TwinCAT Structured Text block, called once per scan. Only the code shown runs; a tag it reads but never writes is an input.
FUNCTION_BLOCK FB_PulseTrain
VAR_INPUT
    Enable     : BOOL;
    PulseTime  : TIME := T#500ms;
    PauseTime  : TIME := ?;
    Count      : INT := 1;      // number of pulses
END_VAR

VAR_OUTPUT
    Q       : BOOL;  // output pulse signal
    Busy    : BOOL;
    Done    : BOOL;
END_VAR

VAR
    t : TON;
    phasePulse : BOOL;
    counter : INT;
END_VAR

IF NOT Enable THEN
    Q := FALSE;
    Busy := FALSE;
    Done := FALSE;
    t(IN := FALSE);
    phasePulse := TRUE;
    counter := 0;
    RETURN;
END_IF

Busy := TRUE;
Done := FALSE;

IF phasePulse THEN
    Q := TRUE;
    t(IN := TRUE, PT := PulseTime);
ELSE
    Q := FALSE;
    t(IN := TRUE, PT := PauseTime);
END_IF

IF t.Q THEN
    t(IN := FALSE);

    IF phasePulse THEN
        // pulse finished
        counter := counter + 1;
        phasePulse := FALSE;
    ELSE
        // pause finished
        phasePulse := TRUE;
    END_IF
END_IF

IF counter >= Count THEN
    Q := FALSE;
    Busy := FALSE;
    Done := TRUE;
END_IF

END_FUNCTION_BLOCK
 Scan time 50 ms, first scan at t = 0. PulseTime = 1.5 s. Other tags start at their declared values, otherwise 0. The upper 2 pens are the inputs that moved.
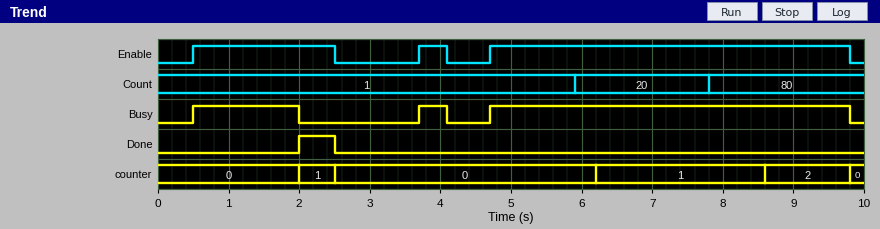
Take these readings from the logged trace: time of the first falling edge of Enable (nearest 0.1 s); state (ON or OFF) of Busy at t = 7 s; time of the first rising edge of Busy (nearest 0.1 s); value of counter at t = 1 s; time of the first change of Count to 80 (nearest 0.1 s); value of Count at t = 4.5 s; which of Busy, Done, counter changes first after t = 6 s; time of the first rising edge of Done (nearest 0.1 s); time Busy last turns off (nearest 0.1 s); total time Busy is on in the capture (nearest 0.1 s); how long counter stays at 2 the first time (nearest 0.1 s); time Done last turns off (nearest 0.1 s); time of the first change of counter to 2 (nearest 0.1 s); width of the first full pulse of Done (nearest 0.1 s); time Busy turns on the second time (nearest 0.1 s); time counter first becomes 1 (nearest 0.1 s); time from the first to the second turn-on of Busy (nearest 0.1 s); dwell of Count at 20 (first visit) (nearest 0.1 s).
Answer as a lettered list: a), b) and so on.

a) 2.5 s
b) ON
c) 0.5 s
d) 0
e) 7.8 s
f) 1
g) counter
h) 2.0 s
i) 9.8 s
j) 7.0 s
k) 1.2 s
l) 2.5 s
m) 8.6 s
n) 0.5 s
o) 3.7 s
p) 2.0 s
q) 3.2 s
r) 1.9 s
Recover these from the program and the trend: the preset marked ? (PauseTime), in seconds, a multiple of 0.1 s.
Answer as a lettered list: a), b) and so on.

a) 0.8 s
